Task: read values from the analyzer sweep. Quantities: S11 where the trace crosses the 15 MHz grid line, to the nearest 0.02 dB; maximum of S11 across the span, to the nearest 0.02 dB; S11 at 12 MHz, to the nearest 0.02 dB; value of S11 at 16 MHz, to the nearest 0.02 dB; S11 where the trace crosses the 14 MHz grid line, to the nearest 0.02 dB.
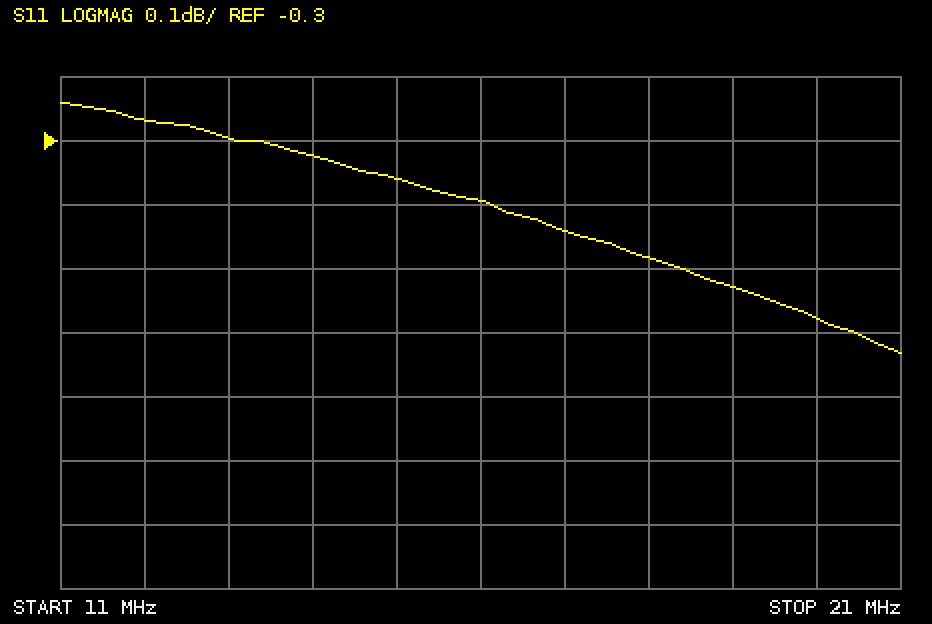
-0.36 dB
-0.24 dB
-0.26 dB
-0.40 dB
-0.32 dB
